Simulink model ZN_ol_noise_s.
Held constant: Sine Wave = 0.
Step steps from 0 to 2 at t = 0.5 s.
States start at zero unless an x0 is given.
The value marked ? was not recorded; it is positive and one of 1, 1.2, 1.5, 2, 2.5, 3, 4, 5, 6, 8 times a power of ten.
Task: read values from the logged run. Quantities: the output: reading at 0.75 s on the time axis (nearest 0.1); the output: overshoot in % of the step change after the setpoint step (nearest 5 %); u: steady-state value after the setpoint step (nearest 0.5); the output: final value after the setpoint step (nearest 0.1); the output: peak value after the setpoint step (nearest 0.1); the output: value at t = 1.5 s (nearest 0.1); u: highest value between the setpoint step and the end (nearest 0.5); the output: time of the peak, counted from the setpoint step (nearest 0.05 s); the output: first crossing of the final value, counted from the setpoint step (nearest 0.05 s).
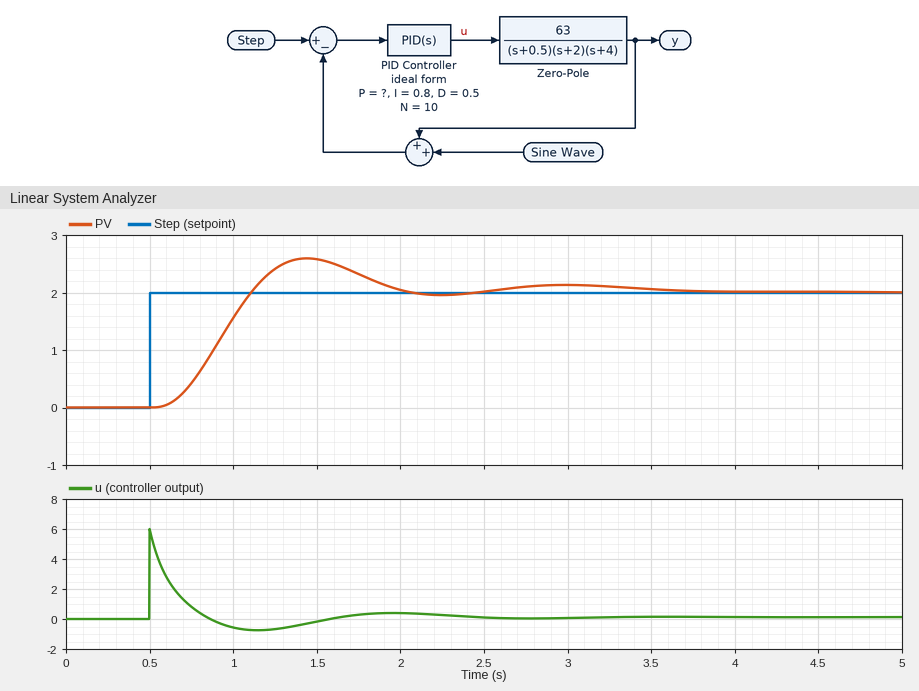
0.4
30 %
0.0
2.0
2.6
2.6
6.0
0.95 s
0.60 s
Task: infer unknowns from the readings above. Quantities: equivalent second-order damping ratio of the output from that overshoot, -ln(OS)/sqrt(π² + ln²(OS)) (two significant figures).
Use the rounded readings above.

0.36
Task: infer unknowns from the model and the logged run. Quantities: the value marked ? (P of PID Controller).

0.5
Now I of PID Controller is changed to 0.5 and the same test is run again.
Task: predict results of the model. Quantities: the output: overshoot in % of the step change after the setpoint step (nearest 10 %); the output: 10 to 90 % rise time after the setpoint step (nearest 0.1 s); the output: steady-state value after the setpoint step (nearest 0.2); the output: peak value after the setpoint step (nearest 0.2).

20 %
0.4 s
2.0
2.4
